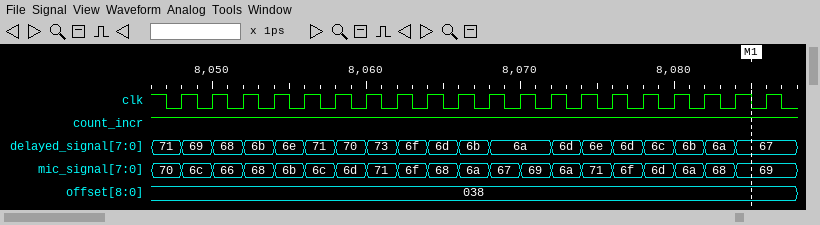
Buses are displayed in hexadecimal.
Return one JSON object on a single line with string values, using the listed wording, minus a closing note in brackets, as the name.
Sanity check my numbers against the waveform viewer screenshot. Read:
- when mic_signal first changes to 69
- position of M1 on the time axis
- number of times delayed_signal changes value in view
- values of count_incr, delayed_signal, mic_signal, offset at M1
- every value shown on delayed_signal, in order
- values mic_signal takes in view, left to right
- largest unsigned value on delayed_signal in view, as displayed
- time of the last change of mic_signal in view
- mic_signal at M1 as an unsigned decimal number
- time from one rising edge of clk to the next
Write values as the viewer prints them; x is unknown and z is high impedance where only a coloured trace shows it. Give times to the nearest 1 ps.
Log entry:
{"when mic_signal first changes to 69": "8070 ps", "position of M1 on the time axis": "8085 ps", "number of times delayed_signal changes value in view": "18", "values of count_incr, delayed_signal, mic_signal, offset at M1": "count_incr=1, delayed_signal=67, mic_signal=69, offset=038", "every value shown on delayed_signal, in order": "71, 69, 68, 6b, 6e, 71, 70, 73, 6f, 6d, 6b, 6a, 6d, 6e, 6d, 6c, 6b, 6a, 67", "values mic_signal takes in view, left to right": "70, 6c, 66, 68, 6b, 6c, 6d, 71, 6f, 68, 6a, 67, 69, 6a, 71, 6f, 6d, 6a, 68, 69", "largest unsigned value on delayed_signal in view, as displayed": "73", "time of the last change of mic_signal in view": "8084 ps", "mic_signal at M1 as an unsigned decimal number": "105", "time from one rising edge of clk to the next": "2 ps"}
